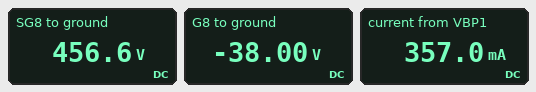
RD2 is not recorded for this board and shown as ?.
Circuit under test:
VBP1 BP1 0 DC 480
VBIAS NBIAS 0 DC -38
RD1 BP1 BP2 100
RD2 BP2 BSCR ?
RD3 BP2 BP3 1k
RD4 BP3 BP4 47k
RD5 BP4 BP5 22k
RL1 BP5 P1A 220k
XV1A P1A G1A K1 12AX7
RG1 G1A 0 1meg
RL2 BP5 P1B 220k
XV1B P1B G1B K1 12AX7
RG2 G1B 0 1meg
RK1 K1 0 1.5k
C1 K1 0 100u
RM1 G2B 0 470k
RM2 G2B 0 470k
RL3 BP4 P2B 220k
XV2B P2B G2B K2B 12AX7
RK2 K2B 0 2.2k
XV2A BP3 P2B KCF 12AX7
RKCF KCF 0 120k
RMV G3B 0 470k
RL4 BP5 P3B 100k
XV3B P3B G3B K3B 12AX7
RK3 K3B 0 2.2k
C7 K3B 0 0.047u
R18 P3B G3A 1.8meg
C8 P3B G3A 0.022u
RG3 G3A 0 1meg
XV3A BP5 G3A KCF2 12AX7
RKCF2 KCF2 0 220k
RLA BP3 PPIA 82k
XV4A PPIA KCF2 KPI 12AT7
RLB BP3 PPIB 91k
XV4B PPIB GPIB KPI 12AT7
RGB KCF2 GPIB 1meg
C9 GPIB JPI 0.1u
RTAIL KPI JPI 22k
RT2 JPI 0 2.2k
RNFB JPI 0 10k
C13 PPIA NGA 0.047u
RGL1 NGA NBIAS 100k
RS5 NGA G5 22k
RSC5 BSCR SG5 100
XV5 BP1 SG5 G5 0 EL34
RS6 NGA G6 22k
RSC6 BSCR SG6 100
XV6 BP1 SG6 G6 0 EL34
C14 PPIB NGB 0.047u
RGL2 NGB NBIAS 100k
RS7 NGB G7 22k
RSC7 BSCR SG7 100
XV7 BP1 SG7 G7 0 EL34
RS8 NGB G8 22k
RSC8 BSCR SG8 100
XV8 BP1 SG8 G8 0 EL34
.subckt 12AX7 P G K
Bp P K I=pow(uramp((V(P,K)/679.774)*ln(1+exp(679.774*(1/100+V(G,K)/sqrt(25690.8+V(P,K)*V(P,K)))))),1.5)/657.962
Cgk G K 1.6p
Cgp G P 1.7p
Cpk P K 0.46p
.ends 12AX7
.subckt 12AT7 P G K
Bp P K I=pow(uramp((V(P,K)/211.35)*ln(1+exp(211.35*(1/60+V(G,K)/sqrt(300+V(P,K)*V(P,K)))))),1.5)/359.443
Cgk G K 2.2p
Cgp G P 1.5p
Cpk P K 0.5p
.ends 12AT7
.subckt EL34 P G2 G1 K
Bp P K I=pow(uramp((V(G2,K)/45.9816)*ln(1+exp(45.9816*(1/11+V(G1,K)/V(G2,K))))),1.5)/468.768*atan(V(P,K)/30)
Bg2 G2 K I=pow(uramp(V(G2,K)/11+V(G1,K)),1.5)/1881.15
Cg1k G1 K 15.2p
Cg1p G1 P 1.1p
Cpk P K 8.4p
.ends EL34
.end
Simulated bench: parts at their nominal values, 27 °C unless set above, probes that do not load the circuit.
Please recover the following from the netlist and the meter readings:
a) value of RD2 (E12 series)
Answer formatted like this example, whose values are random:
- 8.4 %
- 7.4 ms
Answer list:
- 1.5 kΩ
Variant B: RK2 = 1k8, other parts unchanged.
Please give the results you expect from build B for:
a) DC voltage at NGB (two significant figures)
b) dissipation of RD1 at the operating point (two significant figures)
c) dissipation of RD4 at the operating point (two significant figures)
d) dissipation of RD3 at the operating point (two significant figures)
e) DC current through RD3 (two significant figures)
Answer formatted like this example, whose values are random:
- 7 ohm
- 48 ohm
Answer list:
- -38 V
- 46 mW
- 430 mW
- 57 mW
- 7.6 mA
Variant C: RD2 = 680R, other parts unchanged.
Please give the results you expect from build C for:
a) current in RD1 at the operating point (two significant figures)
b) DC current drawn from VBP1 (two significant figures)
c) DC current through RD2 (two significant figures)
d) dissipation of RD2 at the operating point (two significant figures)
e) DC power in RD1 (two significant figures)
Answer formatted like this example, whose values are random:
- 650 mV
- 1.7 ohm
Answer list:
- 26 mA
- 390 mA
- 18 mA
- 230 mW
- 68 mW
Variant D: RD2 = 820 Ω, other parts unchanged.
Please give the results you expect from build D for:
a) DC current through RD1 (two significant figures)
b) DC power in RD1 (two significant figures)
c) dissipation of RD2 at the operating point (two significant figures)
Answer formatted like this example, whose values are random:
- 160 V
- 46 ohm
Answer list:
- 25 mA
- 63 mW
- 250 mW
